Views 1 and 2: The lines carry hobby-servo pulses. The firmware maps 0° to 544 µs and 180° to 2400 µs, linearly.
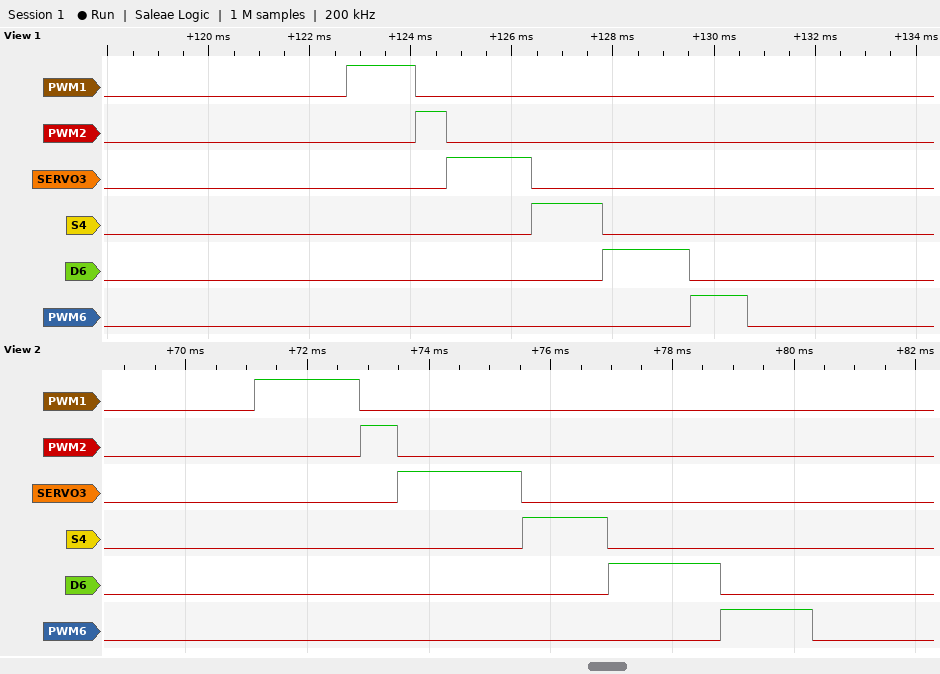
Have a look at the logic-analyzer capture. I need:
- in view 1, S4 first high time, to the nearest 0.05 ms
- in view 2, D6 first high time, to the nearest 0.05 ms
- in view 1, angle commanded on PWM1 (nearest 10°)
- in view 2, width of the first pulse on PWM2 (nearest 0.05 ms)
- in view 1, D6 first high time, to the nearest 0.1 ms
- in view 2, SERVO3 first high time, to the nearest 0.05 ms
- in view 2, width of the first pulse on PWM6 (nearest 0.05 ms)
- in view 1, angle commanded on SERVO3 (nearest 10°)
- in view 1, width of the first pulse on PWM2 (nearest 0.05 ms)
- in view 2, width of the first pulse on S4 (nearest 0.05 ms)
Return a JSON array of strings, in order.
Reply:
["1.40 ms", "1.85 ms", "80°", "0.60 ms", "1.7 ms", "2.05 ms", "1.50 ms", "110°", "0.60 ms", "1.40 ms"]
